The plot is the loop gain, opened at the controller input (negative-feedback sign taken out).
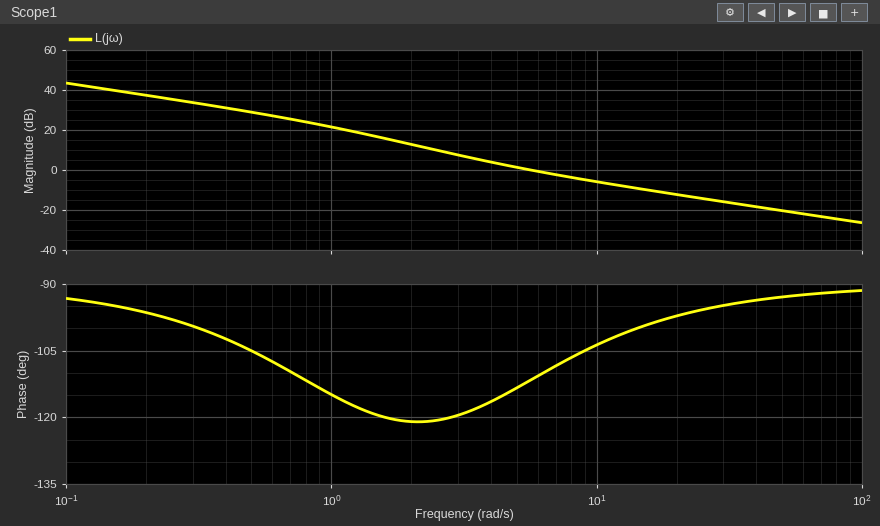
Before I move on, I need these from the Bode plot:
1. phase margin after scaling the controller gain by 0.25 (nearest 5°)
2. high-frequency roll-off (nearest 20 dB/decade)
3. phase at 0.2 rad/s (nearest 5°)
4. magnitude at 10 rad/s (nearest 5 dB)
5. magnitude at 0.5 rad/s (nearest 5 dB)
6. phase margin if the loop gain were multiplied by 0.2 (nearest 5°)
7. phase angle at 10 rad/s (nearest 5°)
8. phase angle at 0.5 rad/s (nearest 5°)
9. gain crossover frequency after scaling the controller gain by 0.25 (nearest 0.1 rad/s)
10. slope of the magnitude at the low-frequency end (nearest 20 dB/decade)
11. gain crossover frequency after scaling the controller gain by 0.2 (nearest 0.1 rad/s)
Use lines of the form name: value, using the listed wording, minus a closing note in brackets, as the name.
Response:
phase margin after scaling the controller gain by 0.25: 60°
high-frequency roll-off: -20 dB/decade
phase at 0.2 rad/s: -95°
magnitude at 10 rad/s: -5 dB
magnitude at 0.5 rad/s: 30 dB
phase margin if the loop gain were multiplied by 0.2: 60°
phase angle at 10 rad/s: -105°
phase angle at 0.5 rad/s: -105°
gain crossover frequency after scaling the controller gain by 0.25: 2.1 rad/s
slope of the magnitude at the low-frequency end: -20 dB/decade
gain crossover frequency after scaling the controller gain by 0.2: 1.8 rad/s
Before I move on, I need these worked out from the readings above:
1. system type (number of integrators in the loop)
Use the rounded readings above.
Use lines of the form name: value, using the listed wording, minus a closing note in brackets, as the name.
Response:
system type: 1
